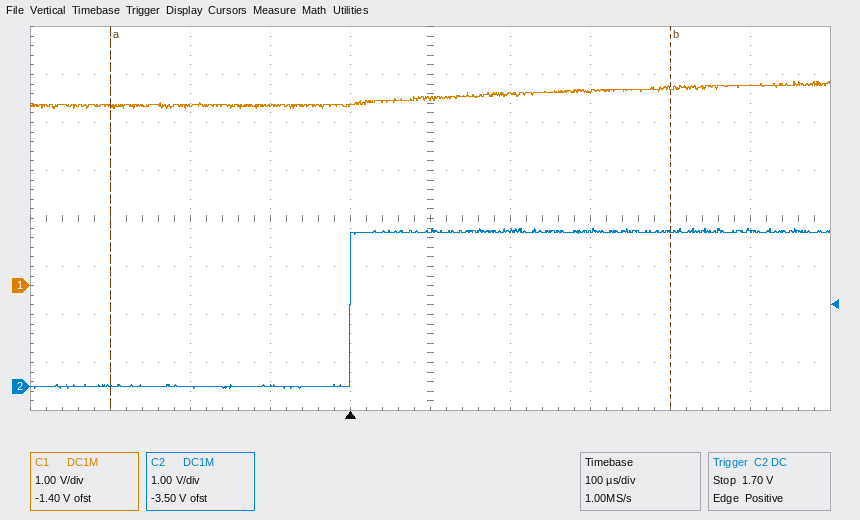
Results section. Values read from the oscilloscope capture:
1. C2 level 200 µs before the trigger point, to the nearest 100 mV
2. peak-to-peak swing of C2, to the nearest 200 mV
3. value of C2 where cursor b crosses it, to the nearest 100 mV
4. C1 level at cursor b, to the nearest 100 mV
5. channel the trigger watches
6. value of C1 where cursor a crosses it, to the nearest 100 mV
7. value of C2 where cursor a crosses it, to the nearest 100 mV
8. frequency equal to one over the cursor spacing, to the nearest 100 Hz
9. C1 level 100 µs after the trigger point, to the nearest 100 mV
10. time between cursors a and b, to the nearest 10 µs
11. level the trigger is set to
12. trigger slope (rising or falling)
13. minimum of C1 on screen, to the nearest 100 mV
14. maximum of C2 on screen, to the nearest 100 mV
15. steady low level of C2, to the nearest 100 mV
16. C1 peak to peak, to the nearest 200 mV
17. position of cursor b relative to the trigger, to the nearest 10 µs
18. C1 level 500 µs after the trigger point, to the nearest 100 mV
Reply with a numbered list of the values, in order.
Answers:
1. 0.0 V
2. 3.4 V
3. 3.2 V
4. 4.1 V
5. C2
6. 3.7 V
7. 0.0 V
8. 1.4 kHz
9. 3.9 V
10. 700 µs
11. 1.70 V
12. rising
13. 3.7 V
14. 3.3 V
15. 0.0 V
16. 600 mV
17. +400 µs
18. 4.2 V
